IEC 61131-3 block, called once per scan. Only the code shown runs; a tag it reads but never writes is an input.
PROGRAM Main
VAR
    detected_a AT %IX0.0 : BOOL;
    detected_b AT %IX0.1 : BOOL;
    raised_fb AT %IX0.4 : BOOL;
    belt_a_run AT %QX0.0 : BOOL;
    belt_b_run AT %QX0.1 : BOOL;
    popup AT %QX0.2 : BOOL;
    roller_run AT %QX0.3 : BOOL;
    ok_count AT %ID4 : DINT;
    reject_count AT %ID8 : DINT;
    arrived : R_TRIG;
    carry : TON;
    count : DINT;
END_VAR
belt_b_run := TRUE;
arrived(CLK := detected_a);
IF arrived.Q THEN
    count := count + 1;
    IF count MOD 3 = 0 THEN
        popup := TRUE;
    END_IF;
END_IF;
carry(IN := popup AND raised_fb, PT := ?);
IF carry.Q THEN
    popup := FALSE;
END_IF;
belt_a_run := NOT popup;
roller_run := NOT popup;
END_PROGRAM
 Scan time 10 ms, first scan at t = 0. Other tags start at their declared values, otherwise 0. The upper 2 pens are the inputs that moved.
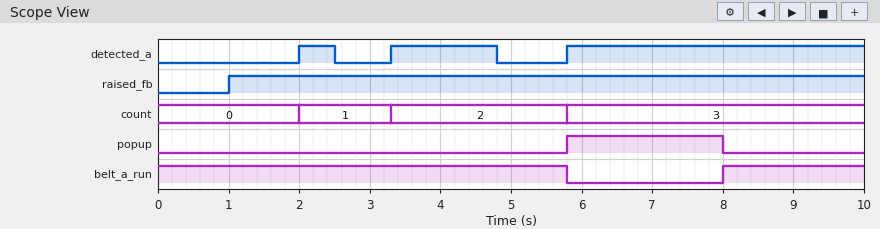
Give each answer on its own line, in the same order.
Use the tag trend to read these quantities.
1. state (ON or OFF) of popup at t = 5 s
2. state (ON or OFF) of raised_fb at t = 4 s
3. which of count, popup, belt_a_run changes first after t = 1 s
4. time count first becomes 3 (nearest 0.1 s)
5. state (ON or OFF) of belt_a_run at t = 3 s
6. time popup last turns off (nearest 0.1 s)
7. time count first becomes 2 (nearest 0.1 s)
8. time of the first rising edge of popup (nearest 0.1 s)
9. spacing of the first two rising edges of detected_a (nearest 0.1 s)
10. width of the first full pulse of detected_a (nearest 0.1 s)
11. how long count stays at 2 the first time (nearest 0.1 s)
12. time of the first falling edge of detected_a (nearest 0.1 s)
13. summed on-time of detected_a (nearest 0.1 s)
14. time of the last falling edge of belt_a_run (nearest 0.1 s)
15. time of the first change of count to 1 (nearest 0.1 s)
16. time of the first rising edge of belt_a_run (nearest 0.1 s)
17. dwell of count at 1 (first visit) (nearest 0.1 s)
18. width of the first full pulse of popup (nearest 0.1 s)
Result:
OFF
ON
count
5.8 s
ON
8.0 s
3.3 s
5.8 s
1.3 s
0.5 s
2.5 s
2.5 s
6.2 s
5.8 s
2.0 s
8.0 s
1.3 s
2.2 s
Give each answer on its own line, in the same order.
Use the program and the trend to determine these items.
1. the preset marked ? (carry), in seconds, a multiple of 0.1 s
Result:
2.2 s
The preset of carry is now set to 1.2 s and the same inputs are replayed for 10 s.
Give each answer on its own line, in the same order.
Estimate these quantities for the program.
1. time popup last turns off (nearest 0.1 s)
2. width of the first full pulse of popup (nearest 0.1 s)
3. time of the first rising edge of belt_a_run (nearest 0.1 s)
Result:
7.0 s
1.2 s
7.0 s
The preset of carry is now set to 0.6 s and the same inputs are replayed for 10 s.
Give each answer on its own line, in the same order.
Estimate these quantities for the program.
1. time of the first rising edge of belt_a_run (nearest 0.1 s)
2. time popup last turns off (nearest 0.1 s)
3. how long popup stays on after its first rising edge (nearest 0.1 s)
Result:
6.4 s
6.4 s
0.6 s
